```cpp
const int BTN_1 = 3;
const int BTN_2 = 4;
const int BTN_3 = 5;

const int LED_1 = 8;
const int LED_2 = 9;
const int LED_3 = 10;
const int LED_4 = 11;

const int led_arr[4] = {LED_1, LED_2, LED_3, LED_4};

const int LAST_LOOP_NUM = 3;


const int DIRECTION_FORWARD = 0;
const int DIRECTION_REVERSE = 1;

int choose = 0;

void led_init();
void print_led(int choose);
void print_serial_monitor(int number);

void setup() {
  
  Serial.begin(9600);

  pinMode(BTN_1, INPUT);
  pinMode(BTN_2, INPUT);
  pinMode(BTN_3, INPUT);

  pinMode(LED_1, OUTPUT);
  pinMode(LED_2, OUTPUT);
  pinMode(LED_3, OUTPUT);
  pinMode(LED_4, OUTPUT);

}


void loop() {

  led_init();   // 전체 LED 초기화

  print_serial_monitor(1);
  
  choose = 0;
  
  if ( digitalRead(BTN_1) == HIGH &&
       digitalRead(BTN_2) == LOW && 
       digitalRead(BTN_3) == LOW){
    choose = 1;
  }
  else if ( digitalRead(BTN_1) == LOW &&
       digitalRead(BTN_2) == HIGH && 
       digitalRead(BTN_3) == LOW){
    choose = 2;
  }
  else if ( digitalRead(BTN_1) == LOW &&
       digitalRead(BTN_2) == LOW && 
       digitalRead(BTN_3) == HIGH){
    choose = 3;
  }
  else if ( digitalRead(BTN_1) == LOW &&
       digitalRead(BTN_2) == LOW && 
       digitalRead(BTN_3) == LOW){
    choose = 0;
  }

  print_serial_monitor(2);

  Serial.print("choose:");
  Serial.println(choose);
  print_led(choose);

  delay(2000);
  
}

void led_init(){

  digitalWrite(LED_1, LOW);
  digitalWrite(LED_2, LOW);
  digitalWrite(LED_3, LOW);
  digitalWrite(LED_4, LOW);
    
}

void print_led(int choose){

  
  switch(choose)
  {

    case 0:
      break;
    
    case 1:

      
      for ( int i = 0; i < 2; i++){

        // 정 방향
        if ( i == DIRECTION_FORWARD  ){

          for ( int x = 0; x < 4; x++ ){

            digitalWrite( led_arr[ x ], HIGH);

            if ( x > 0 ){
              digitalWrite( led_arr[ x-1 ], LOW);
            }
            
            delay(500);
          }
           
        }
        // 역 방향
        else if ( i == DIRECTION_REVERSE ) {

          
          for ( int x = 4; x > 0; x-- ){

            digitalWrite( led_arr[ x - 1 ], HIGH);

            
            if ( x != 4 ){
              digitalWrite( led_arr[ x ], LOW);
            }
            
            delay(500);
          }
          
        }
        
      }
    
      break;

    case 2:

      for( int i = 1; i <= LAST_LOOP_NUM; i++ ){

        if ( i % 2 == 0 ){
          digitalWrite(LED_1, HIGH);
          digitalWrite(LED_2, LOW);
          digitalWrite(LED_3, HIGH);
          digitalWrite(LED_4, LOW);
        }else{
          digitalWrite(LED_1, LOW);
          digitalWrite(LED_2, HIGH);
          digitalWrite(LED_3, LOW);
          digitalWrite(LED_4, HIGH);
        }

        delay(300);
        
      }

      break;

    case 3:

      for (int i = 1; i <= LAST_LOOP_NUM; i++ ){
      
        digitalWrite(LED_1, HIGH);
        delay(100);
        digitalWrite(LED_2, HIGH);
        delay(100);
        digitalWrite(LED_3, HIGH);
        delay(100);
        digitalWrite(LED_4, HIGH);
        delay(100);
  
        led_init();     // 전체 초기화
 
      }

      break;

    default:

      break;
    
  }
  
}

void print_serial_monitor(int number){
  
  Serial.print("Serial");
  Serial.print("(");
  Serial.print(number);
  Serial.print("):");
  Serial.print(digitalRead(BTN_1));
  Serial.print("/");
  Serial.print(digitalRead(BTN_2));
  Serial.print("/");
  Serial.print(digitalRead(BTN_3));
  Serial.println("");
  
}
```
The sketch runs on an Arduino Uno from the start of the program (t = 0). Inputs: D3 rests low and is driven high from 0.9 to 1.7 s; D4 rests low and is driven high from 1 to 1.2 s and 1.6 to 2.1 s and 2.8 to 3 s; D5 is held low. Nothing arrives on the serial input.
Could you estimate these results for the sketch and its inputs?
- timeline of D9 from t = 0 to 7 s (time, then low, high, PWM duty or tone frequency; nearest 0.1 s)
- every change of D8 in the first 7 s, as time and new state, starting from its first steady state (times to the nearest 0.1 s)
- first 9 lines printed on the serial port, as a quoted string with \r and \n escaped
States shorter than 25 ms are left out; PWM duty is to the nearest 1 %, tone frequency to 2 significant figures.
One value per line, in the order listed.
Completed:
0 s low; 2 s high; 2.3 s low; 2.6 s high; 4.9 s low
0 s low; 2.3 s high; 2.6 s low
"Serial(1):0/0/0\r\nSerial(2):0/0/0\r\nchoose:0\r\nSerial(1):0/1/0\r\nSerial(2):0/1/0\r\nchoose:2\r\nSerial(1):0/0/0\r\nSerial(2):0/0/0\r\nchoose:0\r\n"
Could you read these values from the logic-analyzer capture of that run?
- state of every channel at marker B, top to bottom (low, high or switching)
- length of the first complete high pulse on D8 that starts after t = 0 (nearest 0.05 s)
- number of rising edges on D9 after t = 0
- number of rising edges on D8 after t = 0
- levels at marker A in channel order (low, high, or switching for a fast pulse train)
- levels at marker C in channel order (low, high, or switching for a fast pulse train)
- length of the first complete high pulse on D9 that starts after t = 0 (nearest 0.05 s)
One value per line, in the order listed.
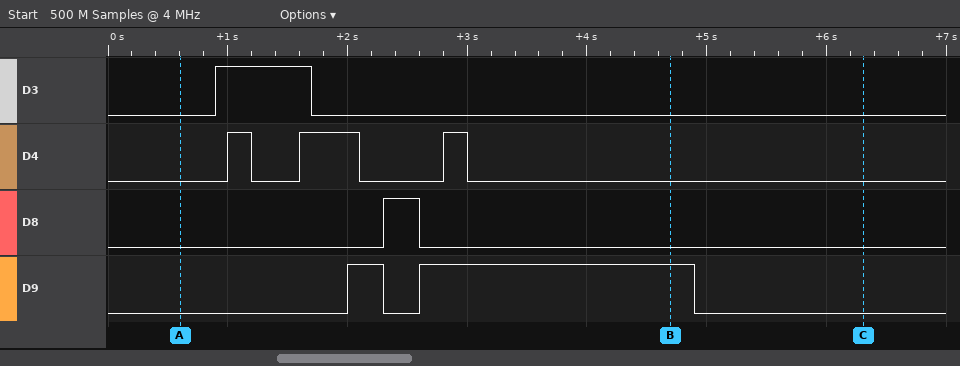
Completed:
D3 low, D4 low, D8 low, D9 high
0.30 s
2
1
D3 low, D4 low, D8 low, D9 low
D3 low, D4 low, D8 low, D9 low
0.30 s
